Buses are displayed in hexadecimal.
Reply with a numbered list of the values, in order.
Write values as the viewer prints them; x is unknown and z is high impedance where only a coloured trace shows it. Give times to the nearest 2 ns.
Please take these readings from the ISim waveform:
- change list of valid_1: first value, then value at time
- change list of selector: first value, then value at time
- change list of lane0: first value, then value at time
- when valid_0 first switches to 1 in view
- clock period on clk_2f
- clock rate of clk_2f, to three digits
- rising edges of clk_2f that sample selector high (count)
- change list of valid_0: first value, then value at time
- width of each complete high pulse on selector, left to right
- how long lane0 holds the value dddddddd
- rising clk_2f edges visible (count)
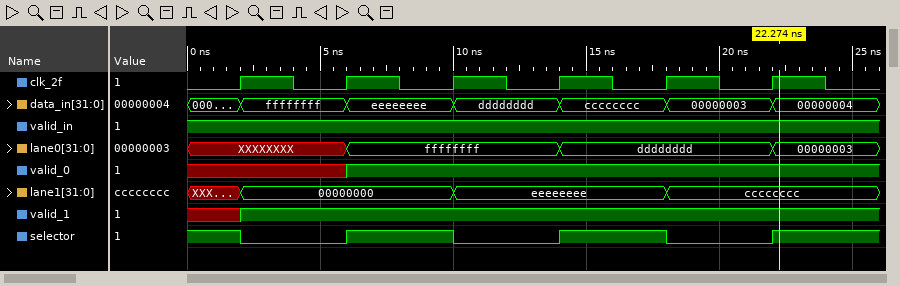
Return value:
1. x, 1 at 2 ns
2. 1, 0 at 2 ns, 1 at 6 ns, 0 at 10 ns, 1 at 14 ns, 0 at 18 ns, 1 at 22 ns
3. XXXXXXXX, ffffffff at 6 ns, dddddddd at 14 ns, 00000003 at 22 ns
4. 6 ns
5. 4 ns
6. 250 MHz
7. 3
8. x, 1 at 6 ns
9. 4 ns, 4 ns
10. 8 ns
11. 6
